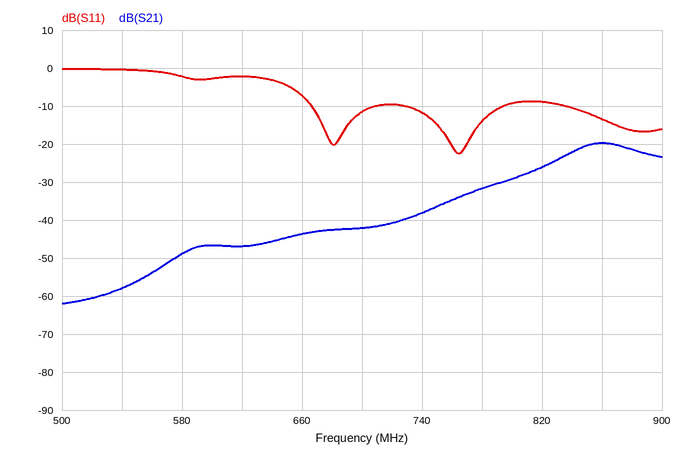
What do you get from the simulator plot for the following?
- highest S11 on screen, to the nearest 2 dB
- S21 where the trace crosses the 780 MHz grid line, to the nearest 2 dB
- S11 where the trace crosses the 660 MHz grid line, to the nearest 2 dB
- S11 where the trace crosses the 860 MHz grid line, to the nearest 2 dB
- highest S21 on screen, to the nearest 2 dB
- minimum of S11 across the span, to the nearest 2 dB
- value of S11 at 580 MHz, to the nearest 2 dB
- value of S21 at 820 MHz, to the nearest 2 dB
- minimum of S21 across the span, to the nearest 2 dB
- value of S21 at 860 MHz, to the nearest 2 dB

0 dB
-32 dB
-8 dB
-14 dB
-20 dB
-22 dB
-2 dB
-26 dB
-62 dB
-20 dB
